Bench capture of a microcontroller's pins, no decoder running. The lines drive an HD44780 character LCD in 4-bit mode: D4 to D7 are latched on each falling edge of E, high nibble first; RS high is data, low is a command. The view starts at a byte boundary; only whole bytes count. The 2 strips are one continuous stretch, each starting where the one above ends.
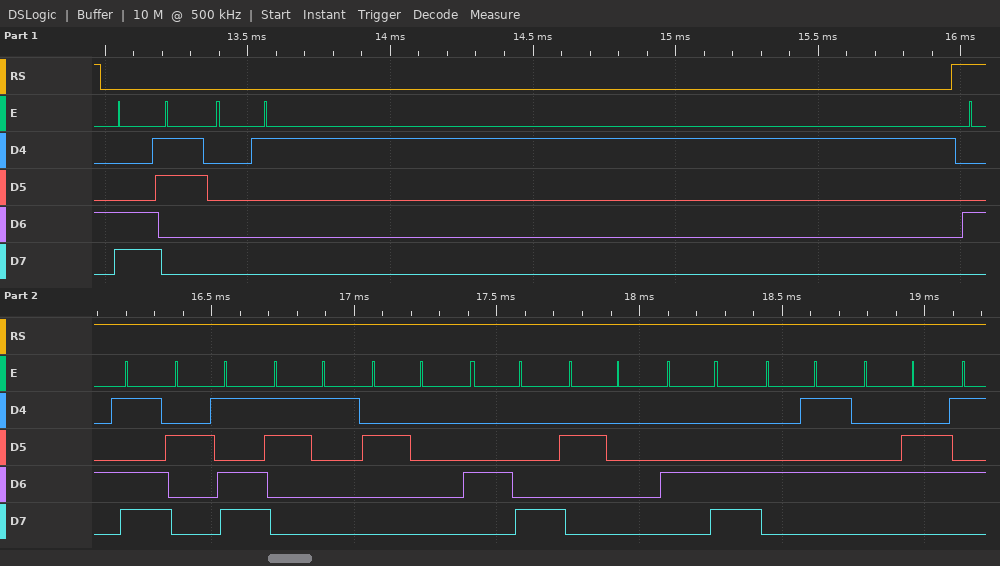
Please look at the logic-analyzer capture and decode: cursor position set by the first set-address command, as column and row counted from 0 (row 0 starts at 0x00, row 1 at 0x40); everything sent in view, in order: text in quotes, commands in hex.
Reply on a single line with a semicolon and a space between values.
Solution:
column 3, row 1; 0xC3 0x01 "M-1 H LEF"
